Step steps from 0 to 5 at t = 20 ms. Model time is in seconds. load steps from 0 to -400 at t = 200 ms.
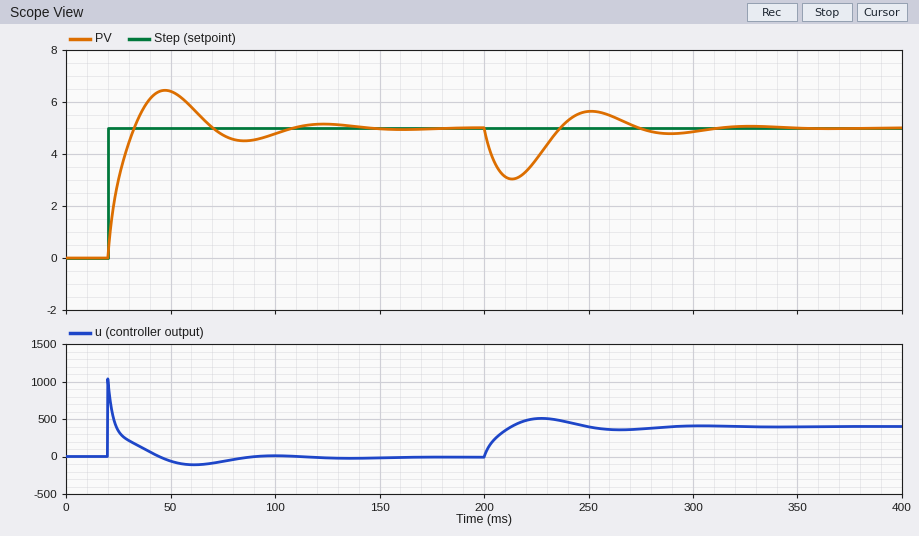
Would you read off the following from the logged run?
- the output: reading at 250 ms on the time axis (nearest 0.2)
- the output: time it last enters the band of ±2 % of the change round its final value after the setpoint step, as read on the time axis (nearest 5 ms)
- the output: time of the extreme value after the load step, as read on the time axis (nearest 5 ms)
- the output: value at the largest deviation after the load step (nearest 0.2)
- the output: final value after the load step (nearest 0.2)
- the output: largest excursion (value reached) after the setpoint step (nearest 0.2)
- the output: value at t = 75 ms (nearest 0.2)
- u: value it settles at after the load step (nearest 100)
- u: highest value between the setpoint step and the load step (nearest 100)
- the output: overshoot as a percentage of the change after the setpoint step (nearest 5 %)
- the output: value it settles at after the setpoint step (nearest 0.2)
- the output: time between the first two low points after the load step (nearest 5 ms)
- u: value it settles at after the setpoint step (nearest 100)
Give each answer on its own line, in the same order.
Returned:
5.6
135 ms
215 ms
3.0
5.0
6.4
4.8
400
1000
30 %
5.0
75 ms
0
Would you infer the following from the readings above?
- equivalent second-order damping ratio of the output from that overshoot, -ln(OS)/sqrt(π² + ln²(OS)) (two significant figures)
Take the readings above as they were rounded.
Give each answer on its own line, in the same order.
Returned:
0.36
